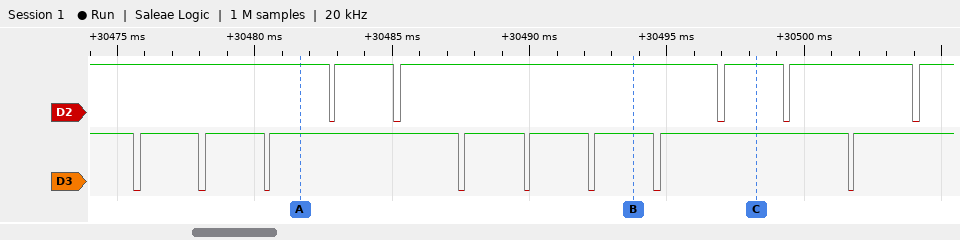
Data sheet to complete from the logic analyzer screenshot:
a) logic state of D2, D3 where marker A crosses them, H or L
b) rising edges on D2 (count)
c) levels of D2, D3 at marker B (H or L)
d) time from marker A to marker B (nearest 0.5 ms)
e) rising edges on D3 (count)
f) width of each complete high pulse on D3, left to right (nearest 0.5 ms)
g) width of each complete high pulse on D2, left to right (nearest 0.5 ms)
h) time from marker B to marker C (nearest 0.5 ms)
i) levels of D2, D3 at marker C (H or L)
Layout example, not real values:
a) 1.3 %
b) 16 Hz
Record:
a) D2=H, D3=H
b) 5
c) D2=H, D3=H
d) 12 ms
e) 8
f) 2 ms, 2 ms, 7 ms, 2 ms, 2 ms, 2 ms, 7 ms
g) 2 ms, 11.5 ms, 2 ms, 4.5 ms
h) 4.5 ms
i) D2=H, D3=H
